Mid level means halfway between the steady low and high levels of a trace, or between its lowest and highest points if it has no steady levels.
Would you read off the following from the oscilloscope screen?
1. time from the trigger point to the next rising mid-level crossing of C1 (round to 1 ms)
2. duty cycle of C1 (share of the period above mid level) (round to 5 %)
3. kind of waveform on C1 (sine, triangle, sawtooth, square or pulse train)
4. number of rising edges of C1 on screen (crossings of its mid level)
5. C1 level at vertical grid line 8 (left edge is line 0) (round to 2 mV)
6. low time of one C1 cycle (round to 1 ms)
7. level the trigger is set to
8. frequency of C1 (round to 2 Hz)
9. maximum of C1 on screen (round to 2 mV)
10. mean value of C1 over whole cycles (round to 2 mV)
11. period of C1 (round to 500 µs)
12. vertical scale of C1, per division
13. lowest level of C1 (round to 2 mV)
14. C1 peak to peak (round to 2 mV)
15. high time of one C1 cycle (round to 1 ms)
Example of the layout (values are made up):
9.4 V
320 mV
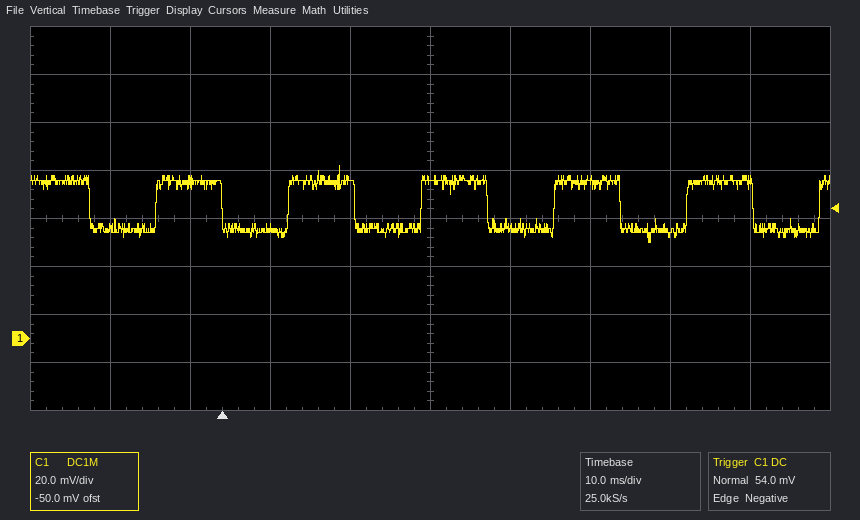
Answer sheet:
8 ms
50 %
square
6
44 mV
8 ms
54.0 mV
60 Hz
72 mV
56 mV
16.5 ms
20 mV
40 mV
32 mV
8 ms
